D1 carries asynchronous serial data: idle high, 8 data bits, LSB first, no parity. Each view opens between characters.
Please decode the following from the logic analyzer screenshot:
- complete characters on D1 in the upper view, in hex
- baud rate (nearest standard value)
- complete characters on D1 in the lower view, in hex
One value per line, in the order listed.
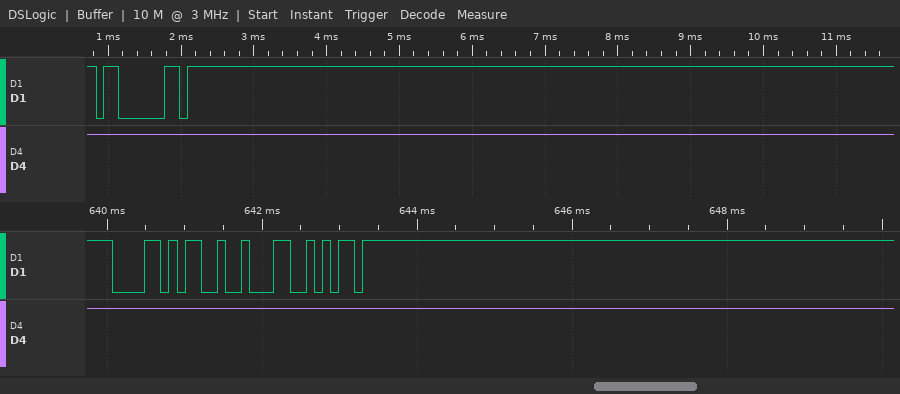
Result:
03, FF
9600 baud
58, 12, 6A
